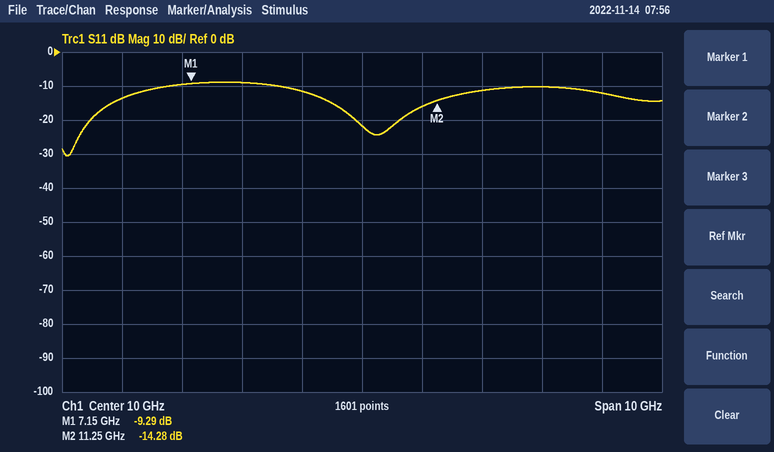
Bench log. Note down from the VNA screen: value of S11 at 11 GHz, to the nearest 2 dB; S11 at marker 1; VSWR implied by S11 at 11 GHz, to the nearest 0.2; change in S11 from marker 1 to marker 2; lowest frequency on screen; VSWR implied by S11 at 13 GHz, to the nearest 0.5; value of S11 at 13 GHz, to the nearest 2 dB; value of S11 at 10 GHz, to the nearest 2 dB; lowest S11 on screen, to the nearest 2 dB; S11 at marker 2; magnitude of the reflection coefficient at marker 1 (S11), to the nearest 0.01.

-16 dB
-9.29 dB
1.4
-4.99 dB
5 GHz
2.0
-10 dB
-22 dB
-30 dB
-14.28 dB
0.34
